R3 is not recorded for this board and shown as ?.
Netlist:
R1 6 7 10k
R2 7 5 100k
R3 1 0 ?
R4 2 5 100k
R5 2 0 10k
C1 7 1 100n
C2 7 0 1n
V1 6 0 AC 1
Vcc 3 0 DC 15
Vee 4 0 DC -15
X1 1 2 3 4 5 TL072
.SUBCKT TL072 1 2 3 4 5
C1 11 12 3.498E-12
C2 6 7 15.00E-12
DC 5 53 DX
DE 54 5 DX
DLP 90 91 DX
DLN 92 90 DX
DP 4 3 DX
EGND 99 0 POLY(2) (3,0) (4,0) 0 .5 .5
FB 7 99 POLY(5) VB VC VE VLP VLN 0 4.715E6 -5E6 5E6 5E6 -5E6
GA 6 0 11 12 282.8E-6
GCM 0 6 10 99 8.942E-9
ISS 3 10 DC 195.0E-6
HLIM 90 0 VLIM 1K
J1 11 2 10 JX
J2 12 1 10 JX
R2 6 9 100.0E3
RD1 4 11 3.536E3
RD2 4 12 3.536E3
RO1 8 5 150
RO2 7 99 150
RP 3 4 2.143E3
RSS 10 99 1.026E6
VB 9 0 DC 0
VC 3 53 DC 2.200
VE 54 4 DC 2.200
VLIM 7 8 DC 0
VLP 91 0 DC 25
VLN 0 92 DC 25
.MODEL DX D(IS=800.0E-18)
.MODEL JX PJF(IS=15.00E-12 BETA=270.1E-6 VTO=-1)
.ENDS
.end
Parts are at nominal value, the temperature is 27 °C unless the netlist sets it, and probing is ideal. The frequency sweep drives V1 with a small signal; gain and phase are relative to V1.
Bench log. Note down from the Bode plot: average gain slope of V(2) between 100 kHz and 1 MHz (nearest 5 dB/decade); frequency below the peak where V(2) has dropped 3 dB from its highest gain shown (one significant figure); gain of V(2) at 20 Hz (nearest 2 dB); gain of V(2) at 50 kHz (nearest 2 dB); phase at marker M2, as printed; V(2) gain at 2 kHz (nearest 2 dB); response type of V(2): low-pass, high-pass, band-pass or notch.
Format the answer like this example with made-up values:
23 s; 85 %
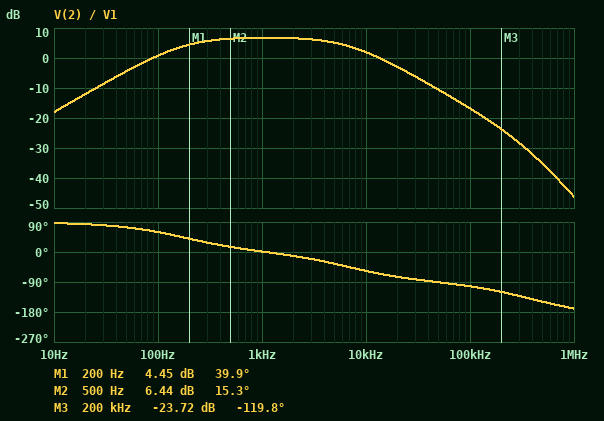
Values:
-30 dB/decade; 200 Hz; -12 dB; -10 dB; 15.3 deg; 6 dB; band-pass
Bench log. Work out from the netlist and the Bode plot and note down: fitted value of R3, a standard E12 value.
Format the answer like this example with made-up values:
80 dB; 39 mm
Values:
22 kΩ
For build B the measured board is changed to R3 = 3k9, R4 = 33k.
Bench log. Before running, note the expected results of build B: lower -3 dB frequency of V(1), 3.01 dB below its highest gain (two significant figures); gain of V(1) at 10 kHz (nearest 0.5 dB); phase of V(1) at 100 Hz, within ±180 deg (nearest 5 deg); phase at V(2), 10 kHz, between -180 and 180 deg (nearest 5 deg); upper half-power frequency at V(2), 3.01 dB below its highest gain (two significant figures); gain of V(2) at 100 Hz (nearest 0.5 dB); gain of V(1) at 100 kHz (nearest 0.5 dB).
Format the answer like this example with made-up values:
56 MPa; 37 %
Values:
140 Hz; -10.5 dB; 55 deg; -10 deg; 51 kHz; -15.0 dB; -17.0 dB
